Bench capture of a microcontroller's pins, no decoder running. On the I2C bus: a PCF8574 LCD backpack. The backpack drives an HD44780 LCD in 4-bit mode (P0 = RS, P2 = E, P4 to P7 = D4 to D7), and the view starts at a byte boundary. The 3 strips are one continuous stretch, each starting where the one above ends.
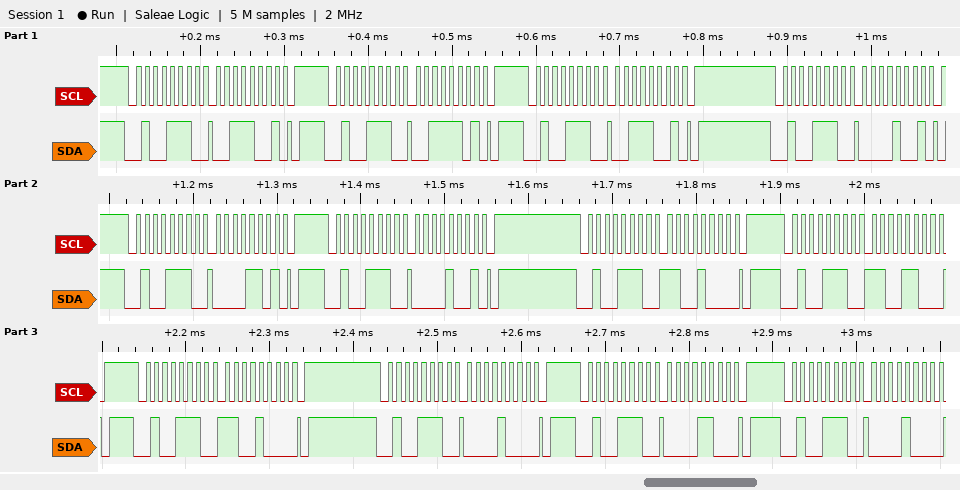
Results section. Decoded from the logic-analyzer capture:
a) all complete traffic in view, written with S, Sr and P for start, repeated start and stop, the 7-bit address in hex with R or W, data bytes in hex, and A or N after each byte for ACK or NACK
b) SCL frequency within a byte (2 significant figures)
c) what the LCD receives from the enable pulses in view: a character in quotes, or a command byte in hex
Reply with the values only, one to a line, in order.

S 27W A 39 A P S 27W A 3D A P S 27W A 39 A P S 27W A 09 A P S 27W A 0D A P S 27W A 09 A P S 27W A C8 A P S 27W A CC A P S 27W A C8 A P S 27W A 08 A P S 27W A 0C A P S 27W A 08 A
100 kHz
'0' 0xC0
